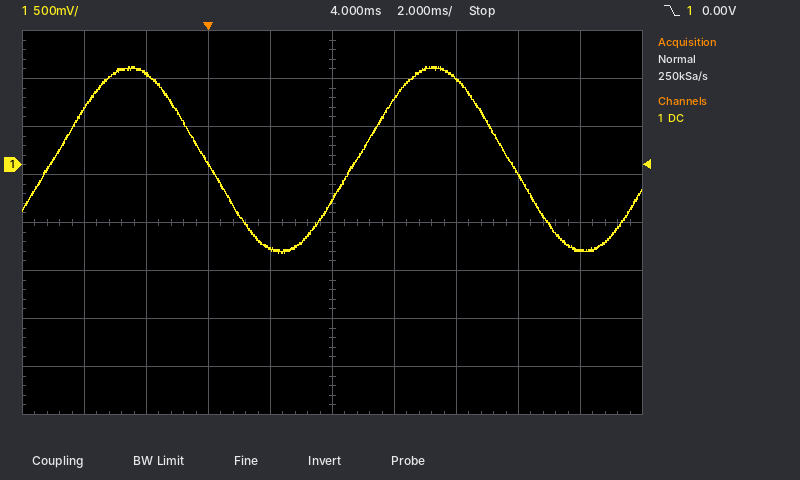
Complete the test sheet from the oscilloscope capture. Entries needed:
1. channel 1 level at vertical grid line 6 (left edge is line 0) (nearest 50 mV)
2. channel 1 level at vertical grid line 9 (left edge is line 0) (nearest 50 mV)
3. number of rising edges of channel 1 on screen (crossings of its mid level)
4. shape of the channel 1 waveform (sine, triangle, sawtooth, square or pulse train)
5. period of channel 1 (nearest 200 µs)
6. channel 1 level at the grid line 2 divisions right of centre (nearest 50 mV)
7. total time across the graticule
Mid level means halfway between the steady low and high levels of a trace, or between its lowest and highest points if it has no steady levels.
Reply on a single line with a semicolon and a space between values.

700 mV; -900 mV; 2; sine; 9.8 ms; 900 mV; 20 ms
